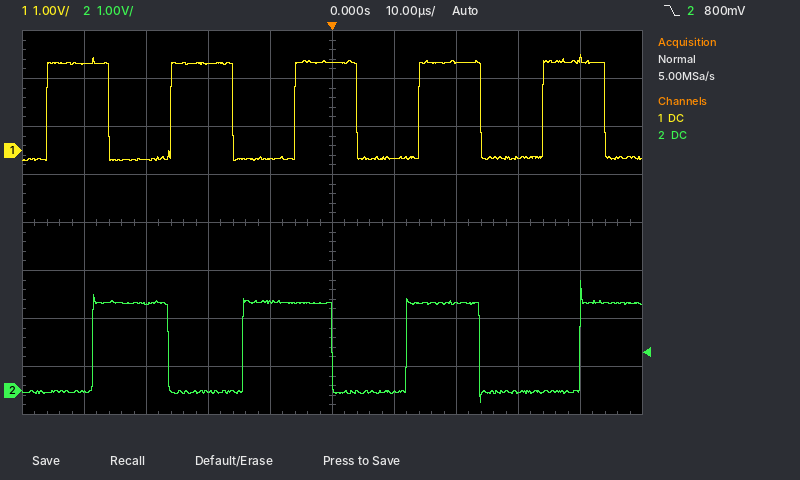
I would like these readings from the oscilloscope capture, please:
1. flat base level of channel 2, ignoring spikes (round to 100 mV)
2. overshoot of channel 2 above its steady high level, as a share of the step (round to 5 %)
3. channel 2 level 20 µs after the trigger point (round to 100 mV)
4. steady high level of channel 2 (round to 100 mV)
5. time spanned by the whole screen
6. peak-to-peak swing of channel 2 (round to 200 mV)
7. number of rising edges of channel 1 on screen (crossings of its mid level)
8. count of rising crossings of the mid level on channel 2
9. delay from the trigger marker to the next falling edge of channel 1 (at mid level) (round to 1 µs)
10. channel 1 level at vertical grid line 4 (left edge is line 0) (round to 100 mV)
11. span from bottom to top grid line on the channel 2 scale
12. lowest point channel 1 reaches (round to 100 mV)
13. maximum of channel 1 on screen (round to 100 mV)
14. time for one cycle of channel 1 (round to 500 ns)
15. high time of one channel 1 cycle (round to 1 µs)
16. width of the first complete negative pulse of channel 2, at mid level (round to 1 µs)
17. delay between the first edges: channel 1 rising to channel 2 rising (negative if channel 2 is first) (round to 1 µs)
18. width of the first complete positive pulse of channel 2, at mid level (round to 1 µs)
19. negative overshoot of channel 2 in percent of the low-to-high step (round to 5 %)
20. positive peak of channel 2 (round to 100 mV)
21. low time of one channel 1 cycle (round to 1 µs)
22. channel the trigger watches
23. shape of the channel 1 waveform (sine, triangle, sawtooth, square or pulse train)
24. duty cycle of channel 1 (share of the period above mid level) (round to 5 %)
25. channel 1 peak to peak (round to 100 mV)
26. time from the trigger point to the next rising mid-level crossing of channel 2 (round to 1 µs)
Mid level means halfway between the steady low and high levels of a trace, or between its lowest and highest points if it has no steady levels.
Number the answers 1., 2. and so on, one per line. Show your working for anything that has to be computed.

1. 0.0 V
2. 25 %
3. 1.8 V
4. 1.8 V
5. 100 µs
6. 2.6 V
7. 5
8. 4
9. 4 µs
10. -200 mV
11. 8 V
12. -200 mV
13. 2.0 V
14. 20.0 µs
15. 10 µs
16. 12 µs
17. +7 µs
18. 12 µs
19. 10 %
20. 2.3 V
21. 10 µs
22. channel 2
23. square
24. 10 µs / 20.0 µs ≈ 50 %
25. 2.0 V − (-200 mV) = 2.2 V
26. 12 µs
